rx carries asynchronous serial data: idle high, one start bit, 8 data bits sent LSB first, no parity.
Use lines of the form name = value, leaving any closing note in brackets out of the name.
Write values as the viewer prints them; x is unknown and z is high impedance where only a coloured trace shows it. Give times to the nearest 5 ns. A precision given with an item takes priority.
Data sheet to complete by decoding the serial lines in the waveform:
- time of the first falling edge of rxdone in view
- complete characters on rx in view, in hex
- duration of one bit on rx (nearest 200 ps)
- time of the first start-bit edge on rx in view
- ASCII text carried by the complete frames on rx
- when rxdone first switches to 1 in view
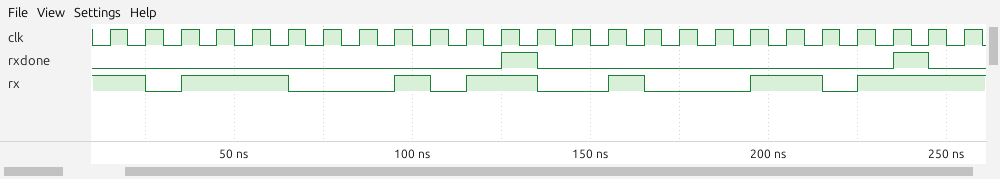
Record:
time of the first falling edge of rxdone in view = 135 ns
complete characters on rx in view, in hex = 47, 62
duration of one bit on rx = 10000 ps
time of the first start-bit edge on rx in view = 25 ns
ASCII text carried by the complete frames on rx = "Gb"
when rxdone first switches to 1 in view = 125 ns
